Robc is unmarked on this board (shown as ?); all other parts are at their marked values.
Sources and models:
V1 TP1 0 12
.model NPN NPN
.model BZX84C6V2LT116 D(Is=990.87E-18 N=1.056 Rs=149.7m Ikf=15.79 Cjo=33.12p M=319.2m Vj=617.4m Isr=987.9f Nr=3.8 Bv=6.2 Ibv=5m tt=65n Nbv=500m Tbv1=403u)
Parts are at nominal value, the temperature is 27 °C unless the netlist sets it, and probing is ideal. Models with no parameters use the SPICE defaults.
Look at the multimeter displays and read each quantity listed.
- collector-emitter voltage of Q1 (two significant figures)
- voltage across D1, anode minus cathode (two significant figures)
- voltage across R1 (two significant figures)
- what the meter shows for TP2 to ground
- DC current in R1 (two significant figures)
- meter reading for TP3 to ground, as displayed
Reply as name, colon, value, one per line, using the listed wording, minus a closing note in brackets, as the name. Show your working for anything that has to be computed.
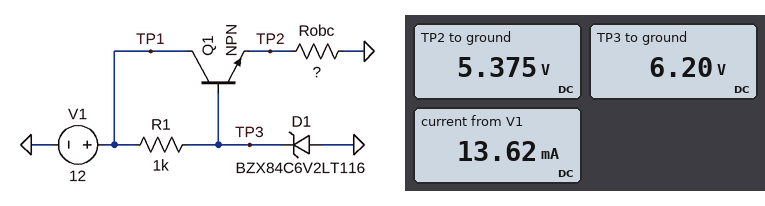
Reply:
collector-emitter voltage of Q1: 12 V - 5.375 V = 6.6 V
voltage across D1, anode minus cathode: 0 V - 6.2 V = -6.2 V
voltage across R1: 12 V - 6.2 V = 5.8 V
what the meter shows for TP2 to ground: 5.375 V
DC current in R1: (12 V - 6.2 V) / 1 kΩ = 5.8 mA
meter reading for TP3 to ground, as displayed: 6.20 V
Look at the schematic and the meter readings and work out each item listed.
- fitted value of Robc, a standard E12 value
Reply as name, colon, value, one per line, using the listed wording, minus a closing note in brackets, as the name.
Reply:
fitted value of Robc, a standard E12 value: 680 Ω
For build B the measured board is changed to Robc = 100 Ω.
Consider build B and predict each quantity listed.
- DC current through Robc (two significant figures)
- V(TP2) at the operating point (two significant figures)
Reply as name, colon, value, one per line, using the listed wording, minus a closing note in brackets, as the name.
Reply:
DC current through Robc: 53 mA
V(TP2) at the operating point: 5.3 V
